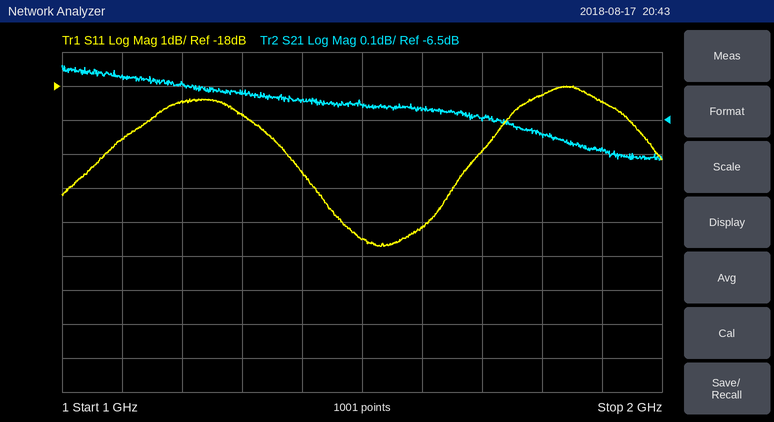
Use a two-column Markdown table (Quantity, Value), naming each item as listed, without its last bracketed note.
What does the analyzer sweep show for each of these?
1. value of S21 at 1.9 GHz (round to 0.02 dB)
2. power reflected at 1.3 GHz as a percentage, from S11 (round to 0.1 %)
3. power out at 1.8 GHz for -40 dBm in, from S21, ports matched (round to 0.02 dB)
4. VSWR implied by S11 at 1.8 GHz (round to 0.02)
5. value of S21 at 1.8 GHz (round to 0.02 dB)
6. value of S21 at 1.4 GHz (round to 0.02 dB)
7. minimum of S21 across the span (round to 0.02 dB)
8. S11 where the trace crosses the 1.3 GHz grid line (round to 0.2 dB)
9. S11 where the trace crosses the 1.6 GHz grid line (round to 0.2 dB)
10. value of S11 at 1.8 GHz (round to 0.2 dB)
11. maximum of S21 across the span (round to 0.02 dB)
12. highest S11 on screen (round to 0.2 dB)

| Quantity | Value |
|---|---|
| value of S21 at 1.9 GHz | -6.58 dB |
| power reflected at 1.3 GHz as a percentage, from S11 | 1.3 % |
| power out at 1.8 GHz for -40 dBm in, from S21, ports matched | -46.54 dBm |
| VSWR implied by S11 at 1.8 GHz | 1.28 |
| value of S21 at 1.8 GHz | -6.54 dB |
| value of S21 at 1.4 GHz | -6.44 dB |
| minimum of S21 across the span | -6.62 dB |
| S11 where the trace crosses the 1.3 GHz grid line | -18.8 dB |
| S11 where the trace crosses the 1.6 GHz grid line | -22.2 dB |
| value of S11 at 1.8 GHz | -18.2 dB |
| maximum of S21 across the span | -6.34 dB |
| highest S11 on screen | -18.0 dB |
